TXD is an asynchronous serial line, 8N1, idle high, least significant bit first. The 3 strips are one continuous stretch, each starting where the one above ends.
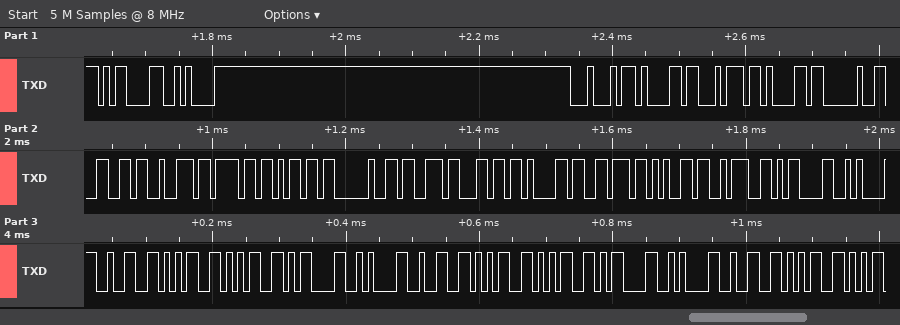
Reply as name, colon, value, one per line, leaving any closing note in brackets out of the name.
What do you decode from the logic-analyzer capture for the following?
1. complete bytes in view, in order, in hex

complete bytes in view, in order, in hex: 0D 0A 44 61 74 61 20 66 72 6F 6D 20 73 6C 61 76 65 3A 0D 0A 32 35 35 0D 0A 32 35 35 0D 0A 32 35
